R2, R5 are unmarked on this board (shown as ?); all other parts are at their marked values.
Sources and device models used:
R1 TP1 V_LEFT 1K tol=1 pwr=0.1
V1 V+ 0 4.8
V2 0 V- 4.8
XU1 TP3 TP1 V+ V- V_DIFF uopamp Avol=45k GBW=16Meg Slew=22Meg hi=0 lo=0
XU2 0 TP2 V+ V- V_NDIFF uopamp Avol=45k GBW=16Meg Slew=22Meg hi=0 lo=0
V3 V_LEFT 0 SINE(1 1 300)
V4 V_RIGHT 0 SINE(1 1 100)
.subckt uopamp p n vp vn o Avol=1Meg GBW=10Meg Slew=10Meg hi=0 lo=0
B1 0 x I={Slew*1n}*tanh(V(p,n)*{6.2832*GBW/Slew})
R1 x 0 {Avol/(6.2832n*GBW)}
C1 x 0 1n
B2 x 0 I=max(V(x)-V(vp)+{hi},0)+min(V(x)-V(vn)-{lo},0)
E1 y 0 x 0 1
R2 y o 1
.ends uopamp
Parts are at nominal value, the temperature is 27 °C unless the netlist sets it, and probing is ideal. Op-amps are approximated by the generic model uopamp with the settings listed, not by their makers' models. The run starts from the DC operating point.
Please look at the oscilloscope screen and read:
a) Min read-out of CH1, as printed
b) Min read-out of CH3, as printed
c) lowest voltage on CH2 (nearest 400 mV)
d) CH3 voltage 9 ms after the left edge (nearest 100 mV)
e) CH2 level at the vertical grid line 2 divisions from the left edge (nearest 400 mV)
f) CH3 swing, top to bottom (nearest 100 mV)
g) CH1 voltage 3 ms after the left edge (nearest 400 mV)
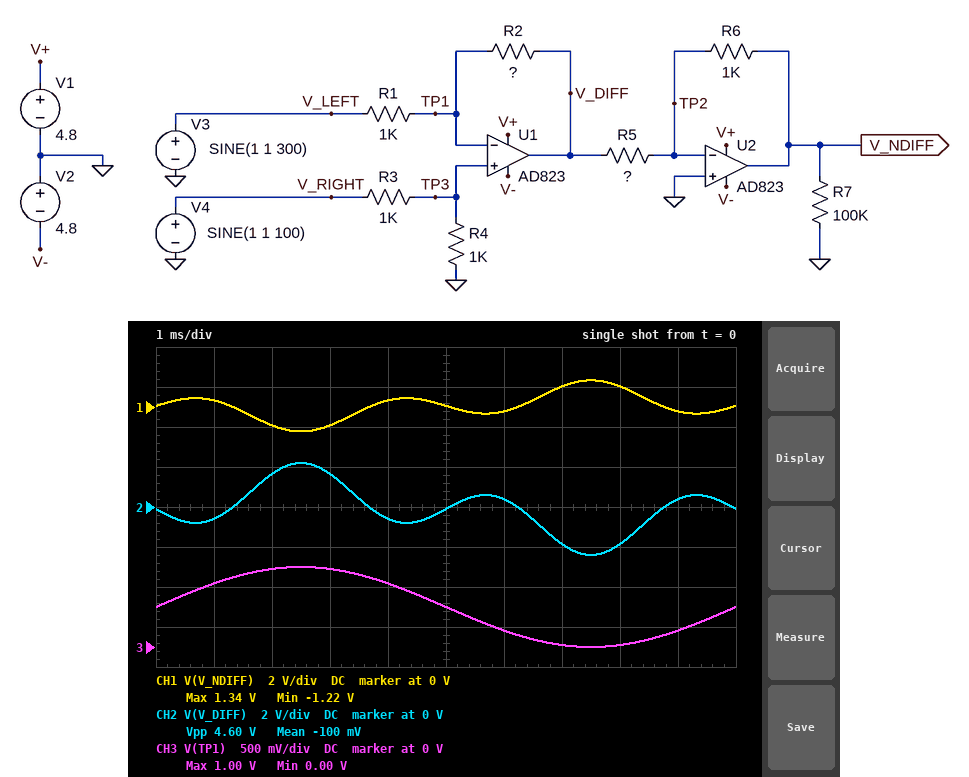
-1.22 V
0.00 V
-2.4 V
200 mV
1.6 V
1.0 V
-800 mV
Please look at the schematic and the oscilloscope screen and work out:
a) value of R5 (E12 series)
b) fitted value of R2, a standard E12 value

1.8 kΩ
1.2 kΩ
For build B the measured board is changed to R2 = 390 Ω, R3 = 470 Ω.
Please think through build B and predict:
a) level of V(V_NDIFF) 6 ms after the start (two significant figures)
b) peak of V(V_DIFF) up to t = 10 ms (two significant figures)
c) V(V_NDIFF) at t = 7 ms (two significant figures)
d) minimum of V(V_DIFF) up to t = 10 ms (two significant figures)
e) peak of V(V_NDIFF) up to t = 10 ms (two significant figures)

-210 mV
1.9 V
320 mV
-780 mV
430 mV
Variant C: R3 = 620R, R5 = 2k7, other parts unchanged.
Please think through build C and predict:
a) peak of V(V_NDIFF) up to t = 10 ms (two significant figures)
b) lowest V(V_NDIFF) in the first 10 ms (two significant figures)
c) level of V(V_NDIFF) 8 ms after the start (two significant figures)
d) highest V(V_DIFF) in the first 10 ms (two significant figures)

890 mV
-1.0 V
680 mV
2.7 V
